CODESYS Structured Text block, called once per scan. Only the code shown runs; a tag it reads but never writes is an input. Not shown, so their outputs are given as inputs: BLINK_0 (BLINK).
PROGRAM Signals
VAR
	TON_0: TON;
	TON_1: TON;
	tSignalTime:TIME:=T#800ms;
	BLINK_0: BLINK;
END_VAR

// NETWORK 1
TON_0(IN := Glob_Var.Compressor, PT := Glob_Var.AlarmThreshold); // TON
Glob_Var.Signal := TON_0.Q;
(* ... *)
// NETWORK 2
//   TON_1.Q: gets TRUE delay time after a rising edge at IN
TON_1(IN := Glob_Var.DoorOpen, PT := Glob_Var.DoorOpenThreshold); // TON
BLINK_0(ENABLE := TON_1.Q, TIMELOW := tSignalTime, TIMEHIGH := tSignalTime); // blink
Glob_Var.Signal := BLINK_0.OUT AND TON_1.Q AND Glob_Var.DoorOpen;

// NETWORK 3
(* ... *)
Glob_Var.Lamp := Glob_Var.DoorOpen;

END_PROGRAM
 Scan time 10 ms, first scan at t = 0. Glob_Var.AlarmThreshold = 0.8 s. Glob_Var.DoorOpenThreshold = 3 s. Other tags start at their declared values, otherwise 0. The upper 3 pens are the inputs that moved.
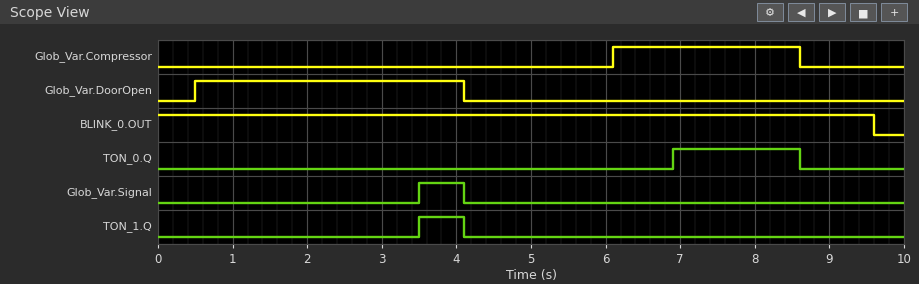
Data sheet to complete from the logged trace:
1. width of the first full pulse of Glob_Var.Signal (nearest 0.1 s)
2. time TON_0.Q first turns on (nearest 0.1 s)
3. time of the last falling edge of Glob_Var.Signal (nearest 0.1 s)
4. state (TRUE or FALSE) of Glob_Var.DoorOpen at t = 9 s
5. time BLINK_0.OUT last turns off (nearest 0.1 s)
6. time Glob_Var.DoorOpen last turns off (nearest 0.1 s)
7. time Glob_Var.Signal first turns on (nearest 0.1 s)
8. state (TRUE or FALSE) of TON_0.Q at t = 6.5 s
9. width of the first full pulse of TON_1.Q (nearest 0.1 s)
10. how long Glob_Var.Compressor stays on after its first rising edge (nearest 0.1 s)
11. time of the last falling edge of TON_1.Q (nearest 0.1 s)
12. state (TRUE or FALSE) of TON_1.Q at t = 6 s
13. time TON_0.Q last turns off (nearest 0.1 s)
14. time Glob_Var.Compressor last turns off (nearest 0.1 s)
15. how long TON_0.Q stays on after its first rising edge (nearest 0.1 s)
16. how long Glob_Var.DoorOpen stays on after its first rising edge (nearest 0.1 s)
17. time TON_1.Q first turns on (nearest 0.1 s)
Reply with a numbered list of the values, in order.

1. 0.6 s
2. 6.9 s
3. 4.1 s
4. FALSE
5. 9.6 s
6. 4.1 s
7. 3.5 s
8. FALSE
9. 0.6 s
10. 2.5 s
11. 4.1 s
12. FALSE
13. 8.6 s
14. 8.6 s
15. 1.7 s
16. 3.6 s
17. 3.5 s
